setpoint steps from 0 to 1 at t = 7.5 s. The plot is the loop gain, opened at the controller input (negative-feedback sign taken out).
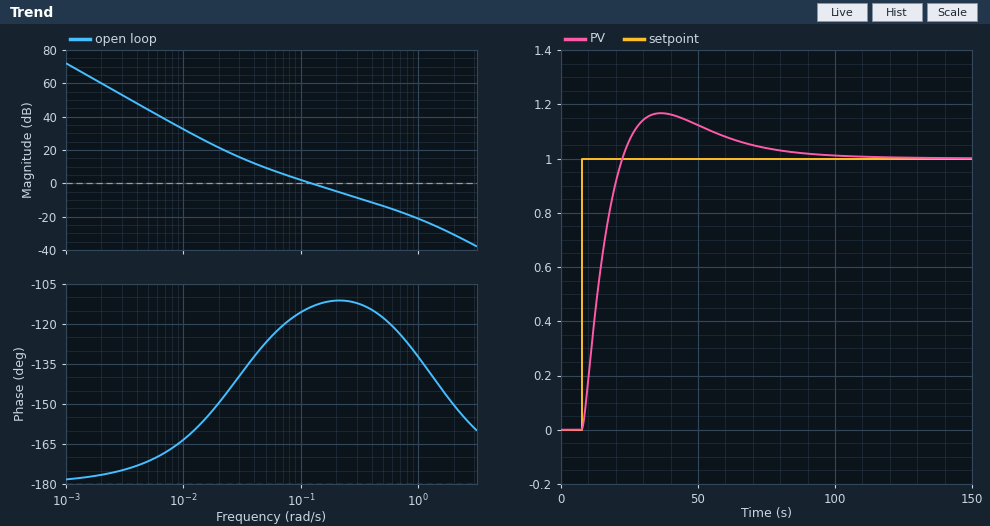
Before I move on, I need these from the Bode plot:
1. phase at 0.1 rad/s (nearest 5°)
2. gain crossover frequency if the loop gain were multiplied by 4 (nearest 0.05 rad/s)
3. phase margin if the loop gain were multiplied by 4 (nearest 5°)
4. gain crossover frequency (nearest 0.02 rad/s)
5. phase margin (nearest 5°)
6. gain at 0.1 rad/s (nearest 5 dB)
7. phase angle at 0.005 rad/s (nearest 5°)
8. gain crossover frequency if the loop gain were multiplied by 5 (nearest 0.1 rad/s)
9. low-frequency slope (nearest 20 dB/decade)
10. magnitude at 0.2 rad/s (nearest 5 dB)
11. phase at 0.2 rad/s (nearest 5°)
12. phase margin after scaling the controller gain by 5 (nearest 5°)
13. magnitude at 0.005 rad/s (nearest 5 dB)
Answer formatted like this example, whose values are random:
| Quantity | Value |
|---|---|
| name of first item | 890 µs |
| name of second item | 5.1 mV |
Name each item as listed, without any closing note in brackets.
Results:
| Quantity | Value |
|---|---|
| phase at 0.1 rad/s | -115° |
| gain crossover frequency if the loop gain were multiplied by 4 | 0.45 rad/s |
| phase margin if the loop gain were multiplied by 4 | 65° |
| gain crossover frequency | 0.12 rad/s |
| phase margin | 65° |
| gain at 0.1 rad/s | 0 dB |
| phase angle at 0.005 rad/s | -170° |
| gain crossover frequency if the loop gain were multiplied by 5 | 0.5 rad/s |
| low-frequency slope | -40 dB/decade |
| magnitude at 0.2 rad/s | -5 dB |
| phase at 0.2 rad/s | -110° |
| phase margin after scaling the controller gain by 5 | 60° |
| magnitude at 0.005 rad/s | 45 dB |
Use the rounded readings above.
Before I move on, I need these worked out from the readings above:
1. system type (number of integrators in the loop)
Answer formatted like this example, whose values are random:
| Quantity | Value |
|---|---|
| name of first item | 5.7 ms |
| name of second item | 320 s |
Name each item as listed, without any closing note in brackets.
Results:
| Quantity | Value |
|---|---|
| system type | 2 |
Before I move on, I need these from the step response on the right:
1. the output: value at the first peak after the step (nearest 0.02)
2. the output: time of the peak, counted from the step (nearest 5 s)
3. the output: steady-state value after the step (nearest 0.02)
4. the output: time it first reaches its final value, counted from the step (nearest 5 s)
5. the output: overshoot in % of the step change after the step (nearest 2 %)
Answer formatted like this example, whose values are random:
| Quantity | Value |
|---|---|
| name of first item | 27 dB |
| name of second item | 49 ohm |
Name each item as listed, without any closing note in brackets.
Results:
| Quantity | Value |
|---|---|
| the output: value at the first peak after the step | 1.16 |
| the output: time of the peak, counted from the step | 30 s |
| the output: steady-state value after the step | 1.00 |
| the output: time it first reaches its final value, counted from the step | 15 s |
| the output: overshoot in % of the step change after the step | 16 % |
